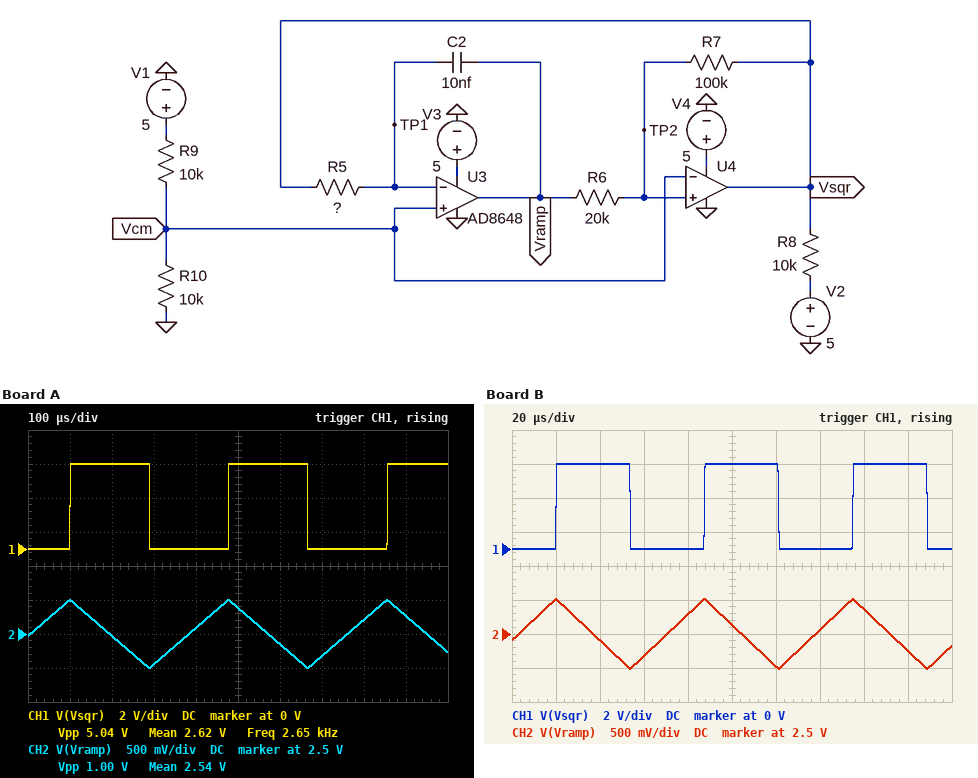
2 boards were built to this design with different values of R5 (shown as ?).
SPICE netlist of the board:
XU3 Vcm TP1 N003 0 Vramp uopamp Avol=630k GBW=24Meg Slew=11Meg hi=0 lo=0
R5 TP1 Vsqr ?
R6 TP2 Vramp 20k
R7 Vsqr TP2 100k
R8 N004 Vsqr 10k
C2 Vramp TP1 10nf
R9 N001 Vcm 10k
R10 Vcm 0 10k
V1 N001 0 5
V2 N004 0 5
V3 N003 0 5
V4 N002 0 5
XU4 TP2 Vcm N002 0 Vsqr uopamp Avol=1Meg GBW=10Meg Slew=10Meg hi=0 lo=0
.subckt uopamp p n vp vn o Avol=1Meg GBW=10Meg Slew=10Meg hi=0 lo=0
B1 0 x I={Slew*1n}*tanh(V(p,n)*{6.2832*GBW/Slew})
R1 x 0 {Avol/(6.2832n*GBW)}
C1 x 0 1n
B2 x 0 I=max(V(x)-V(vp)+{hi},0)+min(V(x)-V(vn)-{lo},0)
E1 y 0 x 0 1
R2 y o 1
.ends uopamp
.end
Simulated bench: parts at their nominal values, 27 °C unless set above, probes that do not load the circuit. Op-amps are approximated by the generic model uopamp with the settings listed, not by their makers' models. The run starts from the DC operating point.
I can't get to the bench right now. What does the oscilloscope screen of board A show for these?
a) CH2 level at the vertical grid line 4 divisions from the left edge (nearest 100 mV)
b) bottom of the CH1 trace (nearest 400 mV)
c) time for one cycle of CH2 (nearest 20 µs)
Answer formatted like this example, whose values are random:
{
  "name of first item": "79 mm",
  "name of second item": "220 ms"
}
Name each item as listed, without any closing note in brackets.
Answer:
{
  "CH2 level at the vertical grid line 4 divisions from the left edge": "2.6 V",
  "bottom of the CH1 trace": "0 V",
  "time for one cycle of CH2": "380 µs"
}
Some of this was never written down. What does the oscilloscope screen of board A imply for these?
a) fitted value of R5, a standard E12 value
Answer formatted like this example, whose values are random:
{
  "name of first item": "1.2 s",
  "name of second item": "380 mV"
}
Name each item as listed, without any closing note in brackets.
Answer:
{
  "fitted value of R5, a standard E12 value": "47 kΩ"
}
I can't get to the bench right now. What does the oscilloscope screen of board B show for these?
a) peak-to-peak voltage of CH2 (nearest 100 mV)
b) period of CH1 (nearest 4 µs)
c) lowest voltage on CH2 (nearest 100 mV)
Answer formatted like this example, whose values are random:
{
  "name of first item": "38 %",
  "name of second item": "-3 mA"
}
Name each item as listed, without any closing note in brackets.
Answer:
{
  "peak-to-peak voltage of CH2": "1.0 V",
  "period of CH1": "68 µs",
  "lowest voltage on CH2": "2.0 V"
}
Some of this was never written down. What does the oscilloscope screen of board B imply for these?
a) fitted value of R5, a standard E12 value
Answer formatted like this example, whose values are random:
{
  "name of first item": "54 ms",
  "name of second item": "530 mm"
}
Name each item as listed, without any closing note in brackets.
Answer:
{
  "fitted value of R5, a standard E12 value": "8.2 kΩ"
}
